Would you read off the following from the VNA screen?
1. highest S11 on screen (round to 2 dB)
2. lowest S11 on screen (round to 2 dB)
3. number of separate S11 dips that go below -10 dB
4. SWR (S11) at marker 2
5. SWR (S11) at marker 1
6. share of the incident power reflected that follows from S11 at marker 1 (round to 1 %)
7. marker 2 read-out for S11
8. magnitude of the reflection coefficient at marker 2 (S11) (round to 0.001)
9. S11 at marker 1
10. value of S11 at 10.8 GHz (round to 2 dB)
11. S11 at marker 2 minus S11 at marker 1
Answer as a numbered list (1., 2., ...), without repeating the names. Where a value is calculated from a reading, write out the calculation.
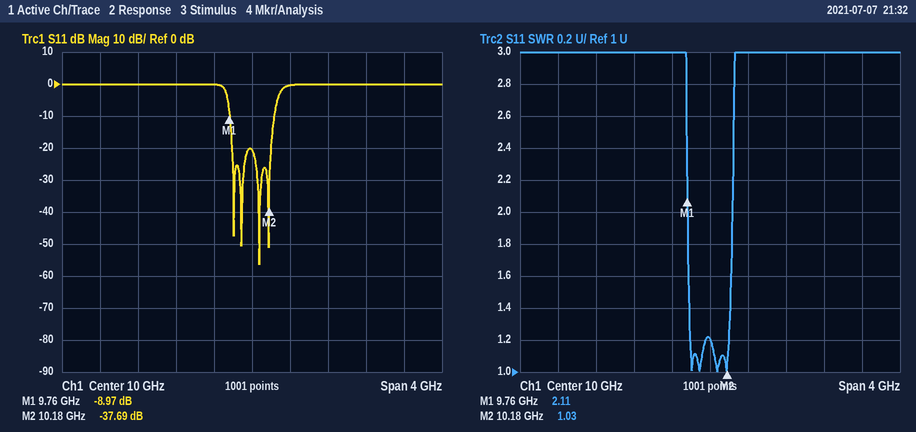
1. 0 dB
2. -56 dB
3. 4
4. 1.03
5. 2.11
6. 10^(-8.97/10) ≈ 13 %
7. -37.69 dB
8. 10^(-37.69/20) ≈ 0.013
9. -8.97 dB
10. 0 dB
11. -37.69 − (-8.97) = -28.72 dB
